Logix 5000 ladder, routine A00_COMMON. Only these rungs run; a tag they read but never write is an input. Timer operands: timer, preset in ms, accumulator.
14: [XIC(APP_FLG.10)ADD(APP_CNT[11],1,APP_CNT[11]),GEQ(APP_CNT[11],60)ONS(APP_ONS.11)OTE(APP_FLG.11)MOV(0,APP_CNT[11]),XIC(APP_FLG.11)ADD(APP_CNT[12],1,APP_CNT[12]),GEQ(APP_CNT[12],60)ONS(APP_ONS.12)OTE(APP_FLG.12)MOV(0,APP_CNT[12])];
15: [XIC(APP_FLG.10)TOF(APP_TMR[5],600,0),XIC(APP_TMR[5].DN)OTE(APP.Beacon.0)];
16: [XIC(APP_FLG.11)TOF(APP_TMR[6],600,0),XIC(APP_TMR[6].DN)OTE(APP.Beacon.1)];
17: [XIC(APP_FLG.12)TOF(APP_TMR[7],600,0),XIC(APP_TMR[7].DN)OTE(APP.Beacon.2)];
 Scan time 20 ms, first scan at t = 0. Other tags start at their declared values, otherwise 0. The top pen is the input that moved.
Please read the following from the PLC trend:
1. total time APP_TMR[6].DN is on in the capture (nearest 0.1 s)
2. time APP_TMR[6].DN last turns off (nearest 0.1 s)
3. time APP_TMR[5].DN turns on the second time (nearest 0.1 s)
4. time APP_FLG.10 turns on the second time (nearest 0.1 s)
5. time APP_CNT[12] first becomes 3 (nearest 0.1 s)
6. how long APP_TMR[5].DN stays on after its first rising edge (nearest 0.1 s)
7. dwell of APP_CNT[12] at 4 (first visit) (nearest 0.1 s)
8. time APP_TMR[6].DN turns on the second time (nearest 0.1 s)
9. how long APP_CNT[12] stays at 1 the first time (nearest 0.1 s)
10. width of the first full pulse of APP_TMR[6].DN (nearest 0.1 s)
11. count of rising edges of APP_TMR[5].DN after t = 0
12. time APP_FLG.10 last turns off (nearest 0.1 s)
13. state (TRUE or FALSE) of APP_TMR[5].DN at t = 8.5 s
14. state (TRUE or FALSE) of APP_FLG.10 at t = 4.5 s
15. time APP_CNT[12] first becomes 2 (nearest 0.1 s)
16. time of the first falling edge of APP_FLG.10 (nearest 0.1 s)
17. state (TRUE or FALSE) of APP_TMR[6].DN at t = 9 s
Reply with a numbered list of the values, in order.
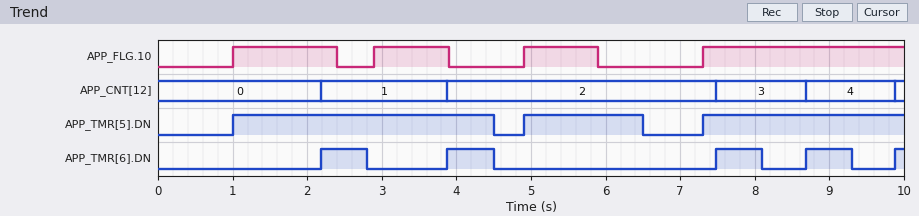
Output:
1. 2.6 s
2. 9.3 s
3. 4.9 s
4. 2.9 s
5. 7.5 s
6. 3.5 s
7. 1.2 s
8. 3.9 s
9. 1.7 s
10. 0.6 s
11. 3
12. 5.9 s
13. TRUE
14. FALSE
15. 3.9 s
16. 2.4 s
17. TRUE
